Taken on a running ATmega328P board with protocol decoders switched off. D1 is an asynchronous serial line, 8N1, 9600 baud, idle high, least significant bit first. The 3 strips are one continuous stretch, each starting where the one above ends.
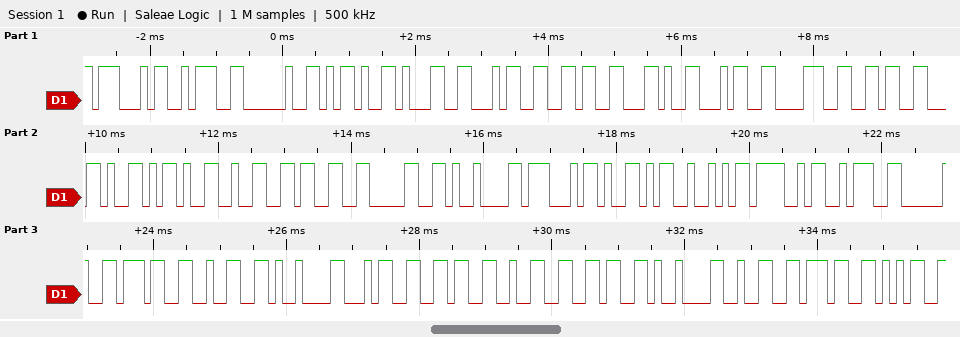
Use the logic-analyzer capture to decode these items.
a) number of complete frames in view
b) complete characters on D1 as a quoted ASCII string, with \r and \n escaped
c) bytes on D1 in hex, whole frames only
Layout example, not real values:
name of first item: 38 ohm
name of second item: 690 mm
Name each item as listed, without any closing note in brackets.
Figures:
number of complete frames in view: 34
complete characters on D1 as a quoted ASCII string, with \r and \n escaped: "G: -146,486,-230\tGYRO: 72\t4626\t275"
bytes on D1 in hex, whole frames only: 47 3A 20 2D 31 34 36 2C 34 38 36 2C 2D 32 33 30 09 47 59 52 4F 3A 20 37 32 09 34 36 32 36 09 32 37 35
